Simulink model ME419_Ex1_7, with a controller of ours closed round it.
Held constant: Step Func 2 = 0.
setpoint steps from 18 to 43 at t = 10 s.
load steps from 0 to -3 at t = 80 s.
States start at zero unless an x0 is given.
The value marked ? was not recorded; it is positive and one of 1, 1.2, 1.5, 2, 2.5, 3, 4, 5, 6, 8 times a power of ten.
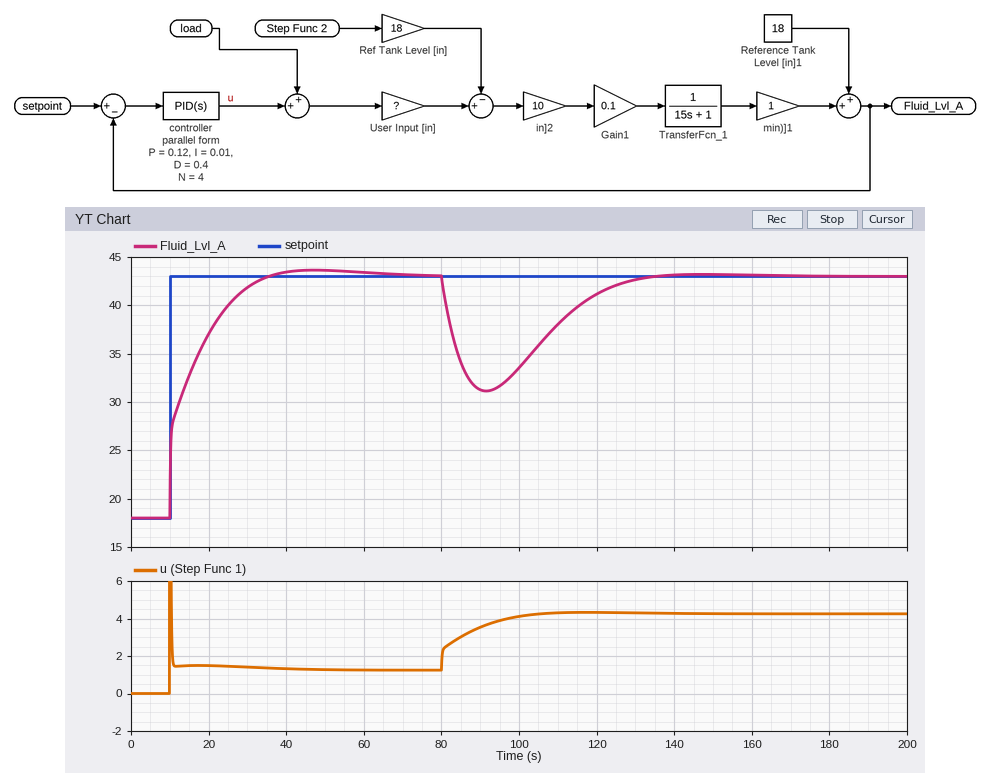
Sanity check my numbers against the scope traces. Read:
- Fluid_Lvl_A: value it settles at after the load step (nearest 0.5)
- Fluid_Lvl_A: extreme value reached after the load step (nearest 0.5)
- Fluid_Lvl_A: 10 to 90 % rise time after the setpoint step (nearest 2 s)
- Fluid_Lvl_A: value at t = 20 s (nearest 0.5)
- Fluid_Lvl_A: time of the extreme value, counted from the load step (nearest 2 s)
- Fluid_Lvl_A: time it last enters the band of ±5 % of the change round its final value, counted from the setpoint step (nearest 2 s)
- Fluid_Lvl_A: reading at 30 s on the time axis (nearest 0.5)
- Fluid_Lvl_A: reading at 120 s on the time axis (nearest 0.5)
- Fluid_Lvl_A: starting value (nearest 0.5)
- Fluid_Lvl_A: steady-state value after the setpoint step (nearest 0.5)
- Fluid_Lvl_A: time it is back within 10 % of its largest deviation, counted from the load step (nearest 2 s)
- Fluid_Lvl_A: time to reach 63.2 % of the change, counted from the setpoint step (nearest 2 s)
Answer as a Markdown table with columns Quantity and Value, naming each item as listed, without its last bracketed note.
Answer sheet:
| Quantity | Value |
|---|---|
| Fluid_Lvl_A: value it settles at after the load step | 43.0 |
| Fluid_Lvl_A: extreme value reached after the load step | 31.0 |
| Fluid_Lvl_A: 10 to 90 % rise time after the setpoint step | 16 s |
| Fluid_Lvl_A: value at t = 20 s | 37.0 |
| Fluid_Lvl_A: time of the extreme value, counted from the load step | 12 s |
| Fluid_Lvl_A: time it last enters the band of ±5 % of the change round its final value, counted from the setpoint step | 20 s |
| Fluid_Lvl_A: reading at 30 s on the time axis | 42.0 |
| Fluid_Lvl_A: reading at 120 s on the time axis | 41.0 |
| Fluid_Lvl_A: starting value | 18.0 |
| Fluid_Lvl_A: steady-state value after the setpoint step | 43.0 |
| Fluid_Lvl_A: time it is back within 10 % of its largest deviation, counted from the load step | 44 s |
| Fluid_Lvl_A: time to reach 63.2 % of the change, counted from the setpoint step | 6 s |
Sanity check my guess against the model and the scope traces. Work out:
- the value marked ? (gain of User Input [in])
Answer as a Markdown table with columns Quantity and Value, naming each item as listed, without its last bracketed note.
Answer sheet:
| Quantity | Value |
|---|---|
| the value marked ? | 20 |
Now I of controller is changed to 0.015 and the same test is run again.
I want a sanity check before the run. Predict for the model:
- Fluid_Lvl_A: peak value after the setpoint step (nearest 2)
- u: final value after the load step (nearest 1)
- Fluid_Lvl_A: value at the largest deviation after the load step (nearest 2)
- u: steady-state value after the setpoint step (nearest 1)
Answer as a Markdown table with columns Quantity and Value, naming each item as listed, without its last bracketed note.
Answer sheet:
| Quantity | Value |
|---|---|
| Fluid_Lvl_A: peak value after the setpoint step | 44 |
| u: final value after the load step | 4 |
| Fluid_Lvl_A: value at the largest deviation after the load step | 32 |
| u: steady-state value after the setpoint step | 1 |
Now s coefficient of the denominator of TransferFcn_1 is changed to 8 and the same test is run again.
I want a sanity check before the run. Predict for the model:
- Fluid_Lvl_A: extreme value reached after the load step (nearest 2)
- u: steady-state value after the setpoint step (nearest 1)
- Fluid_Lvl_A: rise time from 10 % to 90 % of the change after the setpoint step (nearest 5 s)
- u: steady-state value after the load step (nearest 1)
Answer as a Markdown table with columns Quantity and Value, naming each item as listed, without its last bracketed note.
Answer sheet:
| Quantity | Value |
|---|---|
| Fluid_Lvl_A: extreme value reached after the load step | 30 |
| u: steady-state value after the setpoint step | 1 |
| Fluid_Lvl_A: rise time from 10 % to 90 % of the change after the setpoint step | 15 s |
| u: steady-state value after the load step | 4 |
